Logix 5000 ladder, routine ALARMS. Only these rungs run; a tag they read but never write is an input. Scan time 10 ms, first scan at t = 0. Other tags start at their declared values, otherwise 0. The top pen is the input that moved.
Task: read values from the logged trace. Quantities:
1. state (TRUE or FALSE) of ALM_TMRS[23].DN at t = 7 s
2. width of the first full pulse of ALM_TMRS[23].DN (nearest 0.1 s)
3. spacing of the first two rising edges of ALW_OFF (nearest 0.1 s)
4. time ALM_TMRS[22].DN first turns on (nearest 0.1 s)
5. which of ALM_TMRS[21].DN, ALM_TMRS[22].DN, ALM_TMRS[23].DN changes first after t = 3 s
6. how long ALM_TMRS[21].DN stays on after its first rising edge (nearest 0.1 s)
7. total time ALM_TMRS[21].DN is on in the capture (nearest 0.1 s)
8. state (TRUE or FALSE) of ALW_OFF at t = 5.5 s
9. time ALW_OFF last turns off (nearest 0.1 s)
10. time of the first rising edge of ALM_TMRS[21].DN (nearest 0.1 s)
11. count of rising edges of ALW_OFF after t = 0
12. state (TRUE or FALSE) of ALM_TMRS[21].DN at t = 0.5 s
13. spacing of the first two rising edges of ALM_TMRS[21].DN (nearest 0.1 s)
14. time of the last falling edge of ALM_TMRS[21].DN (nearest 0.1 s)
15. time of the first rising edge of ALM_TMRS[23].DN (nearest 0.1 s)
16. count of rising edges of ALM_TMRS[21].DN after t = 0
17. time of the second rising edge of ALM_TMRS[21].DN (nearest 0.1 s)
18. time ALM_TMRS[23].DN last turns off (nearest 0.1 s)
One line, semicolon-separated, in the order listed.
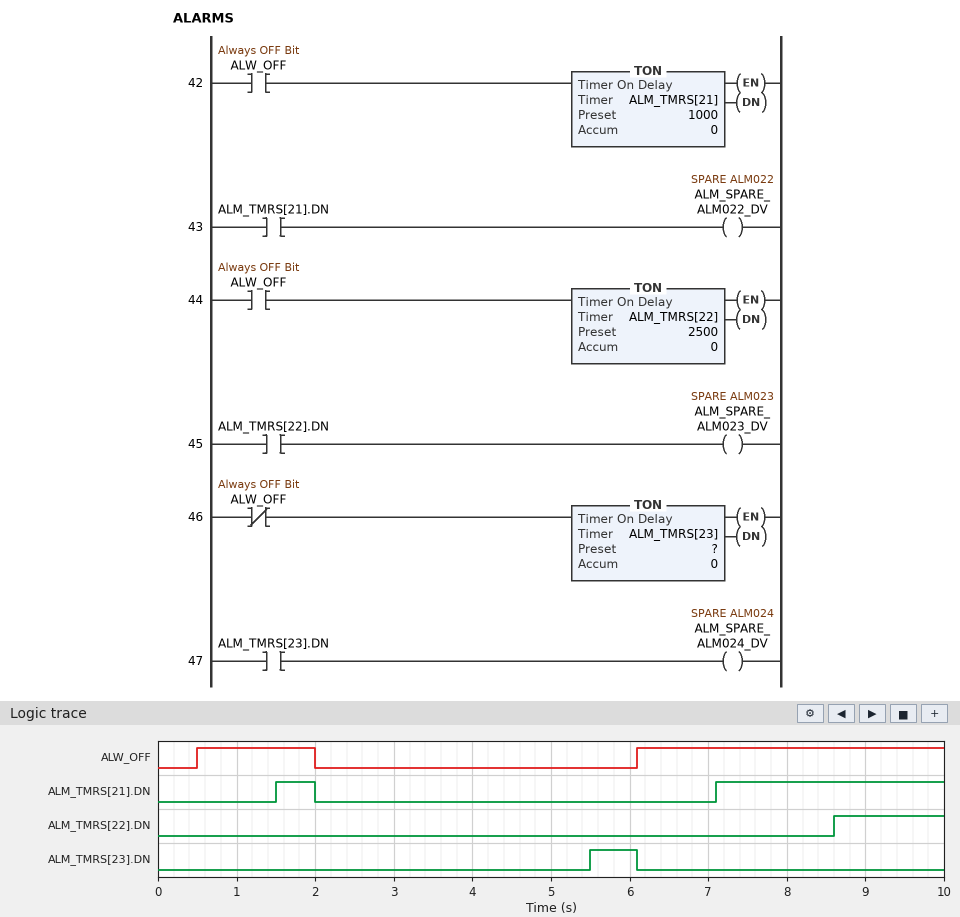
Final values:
FALSE; 0.6 s; 5.6 s; 8.6 s; ALM_TMRS[23].DN; 0.5 s; 3.4 s; FALSE; 2.0 s; 1.5 s; 2; FALSE; 5.6 s; 2.0 s; 5.5 s; 2; 7.1 s; 6.1 s
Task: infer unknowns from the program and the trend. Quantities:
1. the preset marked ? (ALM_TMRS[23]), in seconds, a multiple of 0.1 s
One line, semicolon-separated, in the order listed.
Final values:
3.5 s
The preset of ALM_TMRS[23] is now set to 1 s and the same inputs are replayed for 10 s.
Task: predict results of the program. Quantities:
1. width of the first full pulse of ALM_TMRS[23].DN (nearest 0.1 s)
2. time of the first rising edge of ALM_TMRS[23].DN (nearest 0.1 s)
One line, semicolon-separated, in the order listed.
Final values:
3.1 s; 3.0 s
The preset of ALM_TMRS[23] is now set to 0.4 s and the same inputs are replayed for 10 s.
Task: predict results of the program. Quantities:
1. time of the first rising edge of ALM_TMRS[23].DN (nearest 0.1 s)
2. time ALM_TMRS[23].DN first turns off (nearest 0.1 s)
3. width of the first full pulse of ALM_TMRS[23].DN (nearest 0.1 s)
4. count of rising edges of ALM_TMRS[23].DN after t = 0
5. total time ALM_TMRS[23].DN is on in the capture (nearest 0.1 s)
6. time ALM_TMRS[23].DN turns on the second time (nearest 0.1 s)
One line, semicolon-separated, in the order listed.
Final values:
0.4 s; 0.5 s; 0.1 s; 2; 3.8 s; 2.4 s
